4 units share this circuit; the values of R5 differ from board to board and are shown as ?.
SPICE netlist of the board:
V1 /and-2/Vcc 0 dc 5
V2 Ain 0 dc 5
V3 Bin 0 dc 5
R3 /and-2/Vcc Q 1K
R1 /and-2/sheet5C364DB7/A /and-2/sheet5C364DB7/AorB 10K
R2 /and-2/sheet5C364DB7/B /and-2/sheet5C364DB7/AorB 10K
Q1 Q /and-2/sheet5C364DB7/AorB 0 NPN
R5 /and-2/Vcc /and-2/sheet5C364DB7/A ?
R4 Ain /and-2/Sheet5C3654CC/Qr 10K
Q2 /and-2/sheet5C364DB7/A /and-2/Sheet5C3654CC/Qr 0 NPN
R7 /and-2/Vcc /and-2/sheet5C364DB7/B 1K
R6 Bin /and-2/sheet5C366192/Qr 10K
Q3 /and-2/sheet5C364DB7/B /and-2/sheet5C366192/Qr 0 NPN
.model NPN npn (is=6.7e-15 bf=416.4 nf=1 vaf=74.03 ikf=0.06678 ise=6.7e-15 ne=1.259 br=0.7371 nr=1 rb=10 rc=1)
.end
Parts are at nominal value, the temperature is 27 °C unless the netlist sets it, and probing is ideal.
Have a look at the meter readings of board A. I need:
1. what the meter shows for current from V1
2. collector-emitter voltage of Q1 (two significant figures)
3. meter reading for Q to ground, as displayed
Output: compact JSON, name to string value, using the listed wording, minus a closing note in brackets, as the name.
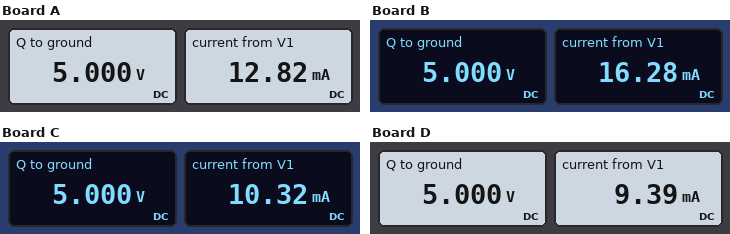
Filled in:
{"what the meter shows for current from V1": "12.82 mA", "collector-emitter voltage of Q1": "5.0 V", "meter reading for Q to ground, as displayed": "5.000 V"}
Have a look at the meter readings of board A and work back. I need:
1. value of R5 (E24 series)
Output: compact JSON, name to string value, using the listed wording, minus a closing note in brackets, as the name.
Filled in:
{"value of R5": "620 Ω"}
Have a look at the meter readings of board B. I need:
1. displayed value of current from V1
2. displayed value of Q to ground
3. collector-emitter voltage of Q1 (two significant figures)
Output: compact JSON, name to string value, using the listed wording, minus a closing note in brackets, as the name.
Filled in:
{"displayed value of current from V1": "16.28 mA", "displayed value of Q to ground": "5.000 V", "collector-emitter voltage of Q1": "5.0 V"}
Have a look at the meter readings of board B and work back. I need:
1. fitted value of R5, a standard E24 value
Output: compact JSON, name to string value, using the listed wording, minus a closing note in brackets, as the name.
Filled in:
{"fitted value of R5, a standard E24 value": "430 Ω"}
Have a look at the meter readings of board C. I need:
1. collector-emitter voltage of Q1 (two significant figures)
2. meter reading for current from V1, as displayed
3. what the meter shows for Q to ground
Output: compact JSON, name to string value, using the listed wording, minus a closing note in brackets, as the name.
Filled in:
{"collector-emitter voltage of Q1": "5.0 V", "meter reading for current from V1, as displayed": "10.32 mA", "what the meter shows for Q to ground": "5.000 V"}
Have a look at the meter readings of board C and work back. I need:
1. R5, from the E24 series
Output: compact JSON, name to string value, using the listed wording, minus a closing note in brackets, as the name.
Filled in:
{"R5, from the E24 series": "910 Ω"}
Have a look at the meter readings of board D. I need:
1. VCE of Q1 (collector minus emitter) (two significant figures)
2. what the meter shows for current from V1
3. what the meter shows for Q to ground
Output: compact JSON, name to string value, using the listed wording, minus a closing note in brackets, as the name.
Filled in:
{"VCE of Q1 (collector minus emitter)": "5.0 V", "what the meter shows for current from V1": "9.39 mA", "what the meter shows for Q to ground": "5.000 V"}
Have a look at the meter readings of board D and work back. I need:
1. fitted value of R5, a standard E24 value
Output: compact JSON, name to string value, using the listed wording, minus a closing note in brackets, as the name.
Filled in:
{"fitted value of R5, a standard E24 value": "1.1 kΩ"}
